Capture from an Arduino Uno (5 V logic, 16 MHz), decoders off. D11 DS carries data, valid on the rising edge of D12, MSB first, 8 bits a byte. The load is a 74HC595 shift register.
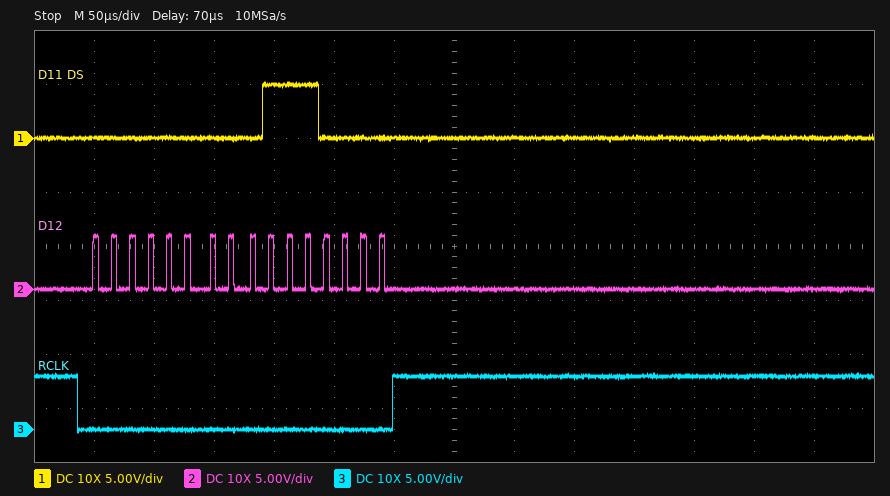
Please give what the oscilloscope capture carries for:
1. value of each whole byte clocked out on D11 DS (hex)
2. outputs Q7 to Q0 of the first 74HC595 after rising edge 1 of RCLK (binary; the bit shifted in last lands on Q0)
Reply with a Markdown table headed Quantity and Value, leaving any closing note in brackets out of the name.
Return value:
| Quantity | Value |
|---|---|
| value of each whole byte clocked out on D11 DS | 0x00 0x70 |
| outputs Q7 to Q0 of the first 74HC595 after rising edge 1 of RCLK | 01110000 |
